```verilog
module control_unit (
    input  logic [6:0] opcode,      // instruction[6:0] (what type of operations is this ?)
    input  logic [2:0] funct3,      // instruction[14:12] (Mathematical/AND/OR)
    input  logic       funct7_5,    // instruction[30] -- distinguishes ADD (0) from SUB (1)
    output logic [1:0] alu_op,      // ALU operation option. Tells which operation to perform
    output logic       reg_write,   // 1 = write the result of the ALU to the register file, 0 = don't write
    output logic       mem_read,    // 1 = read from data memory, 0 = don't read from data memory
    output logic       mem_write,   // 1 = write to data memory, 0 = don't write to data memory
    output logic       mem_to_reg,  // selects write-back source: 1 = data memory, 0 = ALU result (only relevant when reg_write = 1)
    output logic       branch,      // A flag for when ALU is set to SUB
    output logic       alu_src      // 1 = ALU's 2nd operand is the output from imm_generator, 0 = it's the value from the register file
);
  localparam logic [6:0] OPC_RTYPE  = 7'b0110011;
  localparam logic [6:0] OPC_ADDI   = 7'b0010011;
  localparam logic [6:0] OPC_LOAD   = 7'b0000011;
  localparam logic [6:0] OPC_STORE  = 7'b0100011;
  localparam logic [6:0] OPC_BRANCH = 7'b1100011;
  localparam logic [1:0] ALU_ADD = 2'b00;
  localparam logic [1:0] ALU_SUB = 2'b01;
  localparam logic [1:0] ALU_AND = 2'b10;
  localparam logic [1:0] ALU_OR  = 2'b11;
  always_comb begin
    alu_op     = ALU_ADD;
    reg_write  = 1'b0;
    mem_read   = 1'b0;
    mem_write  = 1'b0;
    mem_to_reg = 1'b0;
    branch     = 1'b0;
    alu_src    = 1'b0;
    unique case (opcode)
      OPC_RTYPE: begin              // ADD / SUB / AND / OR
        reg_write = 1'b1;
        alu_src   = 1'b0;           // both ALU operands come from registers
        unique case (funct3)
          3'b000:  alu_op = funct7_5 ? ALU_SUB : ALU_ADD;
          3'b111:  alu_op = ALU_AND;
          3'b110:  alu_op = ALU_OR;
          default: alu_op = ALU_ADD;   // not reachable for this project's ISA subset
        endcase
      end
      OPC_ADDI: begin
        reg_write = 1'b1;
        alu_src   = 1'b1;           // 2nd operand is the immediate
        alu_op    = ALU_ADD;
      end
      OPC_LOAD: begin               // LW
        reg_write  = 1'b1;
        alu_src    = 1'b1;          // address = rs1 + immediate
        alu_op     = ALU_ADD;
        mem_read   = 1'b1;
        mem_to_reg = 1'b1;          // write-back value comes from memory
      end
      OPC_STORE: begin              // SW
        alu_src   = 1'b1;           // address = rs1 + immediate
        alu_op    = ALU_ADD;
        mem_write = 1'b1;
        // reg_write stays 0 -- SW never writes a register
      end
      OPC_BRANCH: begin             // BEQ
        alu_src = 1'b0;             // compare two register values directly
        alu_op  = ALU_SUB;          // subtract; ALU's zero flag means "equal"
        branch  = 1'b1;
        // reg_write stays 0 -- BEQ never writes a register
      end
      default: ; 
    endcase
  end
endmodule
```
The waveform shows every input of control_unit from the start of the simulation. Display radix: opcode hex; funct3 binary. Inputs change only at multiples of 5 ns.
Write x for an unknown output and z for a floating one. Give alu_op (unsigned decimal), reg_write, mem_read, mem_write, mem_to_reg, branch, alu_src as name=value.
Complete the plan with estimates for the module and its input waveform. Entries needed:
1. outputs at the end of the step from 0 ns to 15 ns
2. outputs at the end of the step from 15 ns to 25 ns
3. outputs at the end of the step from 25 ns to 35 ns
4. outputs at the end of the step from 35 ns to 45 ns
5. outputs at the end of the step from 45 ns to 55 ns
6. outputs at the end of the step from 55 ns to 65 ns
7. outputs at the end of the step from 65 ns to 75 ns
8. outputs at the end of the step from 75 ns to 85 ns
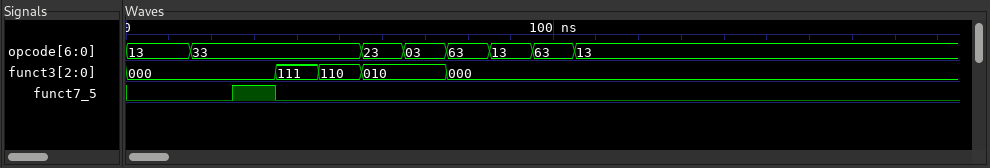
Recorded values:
alu_op=0, reg_write=1, mem_read=0, mem_write=0, mem_to_reg=0, branch=0, alu_src=1
alu_op=0, reg_write=1, mem_read=0, mem_write=0, mem_to_reg=0, branch=0, alu_src=0
alu_op=1, reg_write=1, mem_read=0, mem_write=0, mem_to_reg=0, branch=0, alu_src=0
alu_op=2, reg_write=1, mem_read=0, mem_write=0, mem_to_reg=0, branch=0, alu_src=0
alu_op=3, reg_write=1, mem_read=0, mem_write=0, mem_to_reg=0, branch=0, alu_src=0
alu_op=0, reg_write=0, mem_read=0, mem_write=1, mem_to_reg=0, branch=0, alu_src=1
alu_op=0, reg_write=1, mem_read=1, mem_write=0, mem_to_reg=1, branch=0, alu_src=1
alu_op=1, reg_write=0, mem_read=0, mem_write=0, mem_to_reg=0, branch=1, alu_src=0
